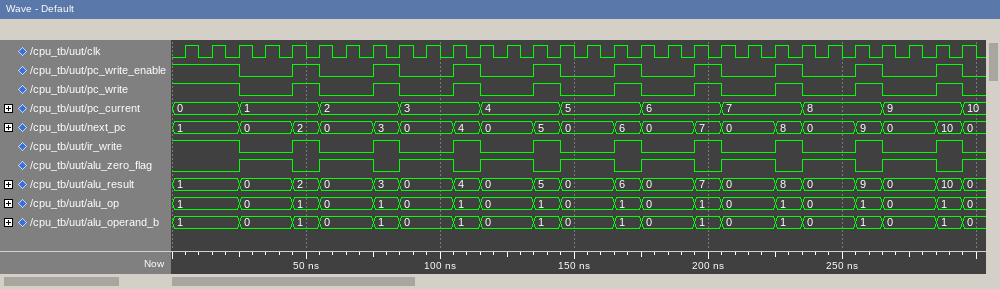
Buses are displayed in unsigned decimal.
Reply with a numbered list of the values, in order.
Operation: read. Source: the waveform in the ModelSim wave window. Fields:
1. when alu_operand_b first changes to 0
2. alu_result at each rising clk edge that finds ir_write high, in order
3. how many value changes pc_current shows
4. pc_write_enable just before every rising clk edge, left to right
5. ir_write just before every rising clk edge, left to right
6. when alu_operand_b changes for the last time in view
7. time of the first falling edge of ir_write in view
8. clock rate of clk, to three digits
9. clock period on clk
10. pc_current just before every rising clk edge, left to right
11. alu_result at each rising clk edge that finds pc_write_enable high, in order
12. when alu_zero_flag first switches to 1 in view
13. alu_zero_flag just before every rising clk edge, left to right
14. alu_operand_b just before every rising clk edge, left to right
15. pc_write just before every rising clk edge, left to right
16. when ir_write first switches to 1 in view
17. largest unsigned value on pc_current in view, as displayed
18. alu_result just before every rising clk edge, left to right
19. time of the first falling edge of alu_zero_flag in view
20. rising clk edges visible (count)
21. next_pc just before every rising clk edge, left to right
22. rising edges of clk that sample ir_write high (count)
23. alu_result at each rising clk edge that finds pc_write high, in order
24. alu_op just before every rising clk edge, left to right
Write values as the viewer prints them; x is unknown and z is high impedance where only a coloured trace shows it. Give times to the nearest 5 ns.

1. 25 ns
2. 1, 1, 1, 2, 3, 4, 5, 6, 7, 8, 9, 10
3. 10
4. 1 1 1 0 0 1 0 0 1 0 0 1 0 0 1 0 0 1 0 0 1 0 0 1 0 0 1 0 0 1
5. 1 1 1 0 0 1 0 0 1 0 0 1 0 0 1 0 0 1 0 0 1 0 0 1 0 0 1 0 0 1
6. 295 ns
7. 25 ns
8. 100 MHz
9. 10 ns
10. 0, 0, 0, 1, 1, 1, 2, 2, 2, 3, 3, 3, 4, 4, 4, 5, 5, 5, 6, 6, 6, 7, 7, 7, 8, 8, 8, 9, 9, 9
11. 1, 1, 1, 2, 3, 4, 5, 6, 7, 8, 9, 10
12. 25 ns
13. 0 0 0 1 1 0 1 1 0 1 1 0 1 1 0 1 1 0 1 1 0 1 1 0 1 1 0 1 1 0
14. 1, 1, 1, 0, 0, 1, 0, 0, 1, 0, 0, 1, 0, 0, 1, 0, 0, 1, 0, 0, 1, 0, 0, 1, 0, 0, 1, 0, 0, 1
15. 1 1 1 0 0 1 0 0 1 0 0 1 0 0 1 0 0 1 0 0 1 0 0 1 0 0 1 0 0 1
16. 45 ns
17. 10
18. 1, 1, 1, 0, 0, 2, 0, 0, 3, 0, 0, 4, 0, 0, 5, 0, 0, 6, 0, 0, 7, 0, 0, 8, 0, 0, 9, 0, 0, 10
19. 45 ns
20. 30
21. 1, 1, 1, 0, 0, 2, 0, 0, 3, 0, 0, 4, 0, 0, 5, 0, 0, 6, 0, 0, 7, 0, 0, 8, 0, 0, 9, 0, 0, 10
22. 12
23. 1, 1, 1, 2, 3, 4, 5, 6, 7, 8, 9, 10
24. 1, 1, 1, 0, 0, 1, 0, 0, 1, 0, 0, 1, 0, 0, 1, 0, 0, 1, 0, 0, 1, 0, 0, 1, 0, 0, 1, 0, 0, 1
